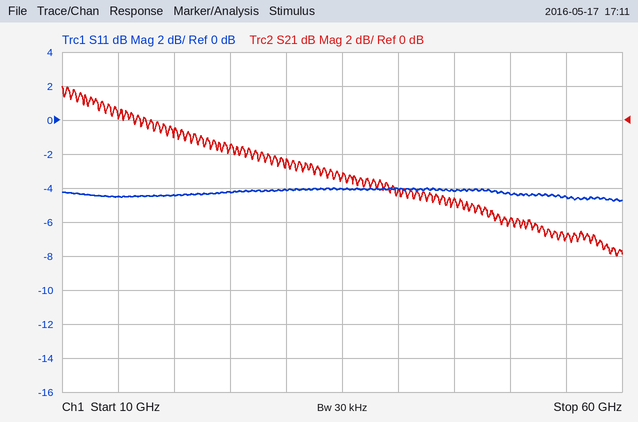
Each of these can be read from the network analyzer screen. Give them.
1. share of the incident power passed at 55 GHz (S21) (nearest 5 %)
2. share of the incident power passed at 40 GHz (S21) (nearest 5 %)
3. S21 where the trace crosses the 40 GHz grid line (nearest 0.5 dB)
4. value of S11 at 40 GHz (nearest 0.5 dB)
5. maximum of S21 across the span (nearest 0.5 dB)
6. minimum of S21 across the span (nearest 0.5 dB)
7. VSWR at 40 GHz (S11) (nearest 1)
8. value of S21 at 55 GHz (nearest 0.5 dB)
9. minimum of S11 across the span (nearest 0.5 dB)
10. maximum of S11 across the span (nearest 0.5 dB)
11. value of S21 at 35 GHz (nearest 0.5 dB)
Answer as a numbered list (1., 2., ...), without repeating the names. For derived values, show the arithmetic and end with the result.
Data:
1. 10^(-7/10) ≈ 20 %
2. 10^(-4/10) ≈ 40 %
3. -4.0 dB
4. -4.0 dB
5. 2.0 dB
6. -8.0 dB
7. |Γ| = 10^(-4/20) = 0.6310; VSWR = (1 + 0.6310)/(1 − 0.6310) ≈ 4
8. -7.0 dB
9. -5.0 dB
10. -4.0 dB
11. -3.5 dB
